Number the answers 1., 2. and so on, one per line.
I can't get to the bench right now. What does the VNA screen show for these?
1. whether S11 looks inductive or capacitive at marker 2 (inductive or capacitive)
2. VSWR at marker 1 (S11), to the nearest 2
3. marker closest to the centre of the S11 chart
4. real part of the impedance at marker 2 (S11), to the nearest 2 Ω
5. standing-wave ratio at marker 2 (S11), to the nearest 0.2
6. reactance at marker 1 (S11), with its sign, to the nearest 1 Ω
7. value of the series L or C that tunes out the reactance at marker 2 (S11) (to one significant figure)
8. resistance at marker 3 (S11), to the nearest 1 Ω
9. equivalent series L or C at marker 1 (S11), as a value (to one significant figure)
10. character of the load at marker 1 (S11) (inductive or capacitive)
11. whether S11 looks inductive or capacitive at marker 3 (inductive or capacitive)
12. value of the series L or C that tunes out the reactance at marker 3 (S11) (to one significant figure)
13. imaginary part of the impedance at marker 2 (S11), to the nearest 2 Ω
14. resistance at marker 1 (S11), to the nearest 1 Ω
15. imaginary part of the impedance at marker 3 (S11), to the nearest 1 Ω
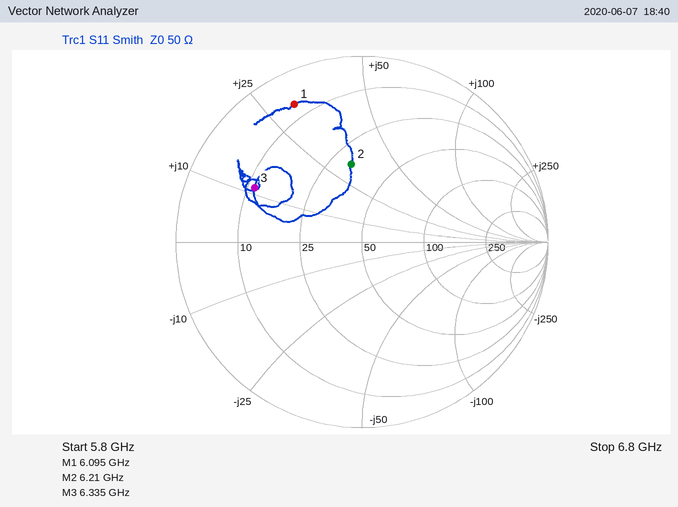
1. inductive
2. 10
3. marker 2
4. 32 Ω
5. 2.4
6. +31 Ω
7. 800 fF
8. 11 Ω
9. 800 pH
10. inductive
11. inductive
12. 2 pF
13. +32 Ω
14. 7 Ω
15. +11 Ω
